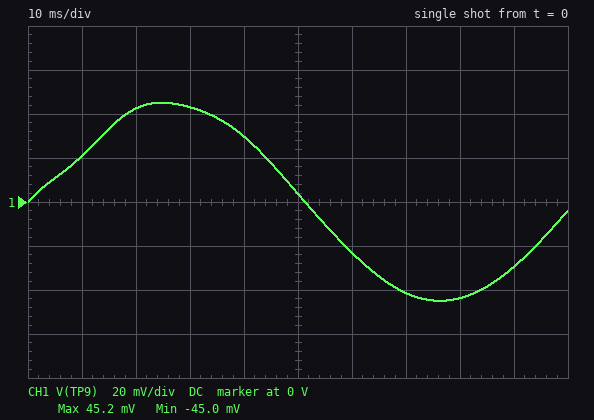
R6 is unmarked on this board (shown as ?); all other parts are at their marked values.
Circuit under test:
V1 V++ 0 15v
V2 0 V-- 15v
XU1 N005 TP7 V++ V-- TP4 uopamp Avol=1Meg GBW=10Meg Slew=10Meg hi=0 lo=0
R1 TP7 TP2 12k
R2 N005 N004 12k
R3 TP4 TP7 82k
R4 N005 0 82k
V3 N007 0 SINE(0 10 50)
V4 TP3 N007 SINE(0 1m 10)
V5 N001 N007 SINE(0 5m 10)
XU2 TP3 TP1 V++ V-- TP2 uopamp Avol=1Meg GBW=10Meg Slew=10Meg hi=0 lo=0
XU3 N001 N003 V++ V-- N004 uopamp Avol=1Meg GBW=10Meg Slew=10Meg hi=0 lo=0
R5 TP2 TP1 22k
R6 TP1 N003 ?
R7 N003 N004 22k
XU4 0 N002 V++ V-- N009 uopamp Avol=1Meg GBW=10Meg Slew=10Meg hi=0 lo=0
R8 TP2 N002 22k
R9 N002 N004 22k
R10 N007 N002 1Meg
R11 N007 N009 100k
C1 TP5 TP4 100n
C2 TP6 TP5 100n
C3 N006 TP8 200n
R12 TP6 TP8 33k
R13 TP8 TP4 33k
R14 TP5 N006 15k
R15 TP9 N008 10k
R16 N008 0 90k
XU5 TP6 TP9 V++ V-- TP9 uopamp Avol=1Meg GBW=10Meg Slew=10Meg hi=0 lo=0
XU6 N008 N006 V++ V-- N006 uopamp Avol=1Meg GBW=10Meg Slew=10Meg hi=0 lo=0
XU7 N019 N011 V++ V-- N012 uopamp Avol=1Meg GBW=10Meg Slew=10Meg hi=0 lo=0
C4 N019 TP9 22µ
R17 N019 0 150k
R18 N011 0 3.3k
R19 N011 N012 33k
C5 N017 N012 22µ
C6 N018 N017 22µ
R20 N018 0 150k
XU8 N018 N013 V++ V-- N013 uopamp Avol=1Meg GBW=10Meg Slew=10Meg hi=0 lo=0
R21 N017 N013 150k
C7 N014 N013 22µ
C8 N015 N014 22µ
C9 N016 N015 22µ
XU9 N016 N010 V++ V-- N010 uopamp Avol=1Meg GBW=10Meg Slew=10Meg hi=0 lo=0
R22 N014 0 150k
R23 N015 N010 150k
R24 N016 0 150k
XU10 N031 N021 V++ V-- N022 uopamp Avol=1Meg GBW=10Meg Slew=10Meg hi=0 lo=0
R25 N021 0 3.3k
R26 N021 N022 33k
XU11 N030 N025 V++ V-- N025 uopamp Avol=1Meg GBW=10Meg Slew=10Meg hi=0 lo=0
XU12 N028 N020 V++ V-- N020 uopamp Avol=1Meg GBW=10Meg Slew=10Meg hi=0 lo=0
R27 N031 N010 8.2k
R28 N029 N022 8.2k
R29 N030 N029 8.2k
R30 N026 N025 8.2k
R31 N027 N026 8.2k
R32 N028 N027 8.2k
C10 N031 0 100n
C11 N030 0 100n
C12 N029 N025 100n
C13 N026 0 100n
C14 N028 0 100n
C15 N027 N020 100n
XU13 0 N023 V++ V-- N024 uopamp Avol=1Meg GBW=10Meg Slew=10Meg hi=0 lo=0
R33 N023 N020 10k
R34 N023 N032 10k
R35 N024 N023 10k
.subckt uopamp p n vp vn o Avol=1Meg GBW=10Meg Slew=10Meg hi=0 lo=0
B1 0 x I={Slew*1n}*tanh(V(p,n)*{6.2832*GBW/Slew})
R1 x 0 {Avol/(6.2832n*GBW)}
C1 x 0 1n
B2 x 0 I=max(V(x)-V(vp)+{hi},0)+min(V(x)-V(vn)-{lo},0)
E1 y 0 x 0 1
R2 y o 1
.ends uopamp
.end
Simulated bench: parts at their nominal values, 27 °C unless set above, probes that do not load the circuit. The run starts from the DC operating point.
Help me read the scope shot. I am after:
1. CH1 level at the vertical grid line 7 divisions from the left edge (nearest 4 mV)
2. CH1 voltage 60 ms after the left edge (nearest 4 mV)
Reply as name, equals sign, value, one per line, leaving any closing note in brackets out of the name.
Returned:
CH1 level at the vertical grid line 7 divisions from the left edge = -40 mV
CH1 voltage 60 ms after the left edge = -24 mV
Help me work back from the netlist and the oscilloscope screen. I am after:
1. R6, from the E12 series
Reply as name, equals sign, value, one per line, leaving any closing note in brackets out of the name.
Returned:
R6, from the E12 series = 68 kΩ
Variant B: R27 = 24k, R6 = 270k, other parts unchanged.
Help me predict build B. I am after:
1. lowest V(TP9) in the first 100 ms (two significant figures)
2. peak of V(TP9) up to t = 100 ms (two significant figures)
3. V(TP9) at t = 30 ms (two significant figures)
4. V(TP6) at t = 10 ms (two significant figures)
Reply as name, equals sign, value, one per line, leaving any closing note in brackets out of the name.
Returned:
lowest V(TP9) in the first 100 ms = -32 mV
peak of V(TP9) up to t = 100 ms = 32 mV
V(TP9) at t = 30 ms = 30 mV
V(TP6) at t = 10 ms = 15 mV
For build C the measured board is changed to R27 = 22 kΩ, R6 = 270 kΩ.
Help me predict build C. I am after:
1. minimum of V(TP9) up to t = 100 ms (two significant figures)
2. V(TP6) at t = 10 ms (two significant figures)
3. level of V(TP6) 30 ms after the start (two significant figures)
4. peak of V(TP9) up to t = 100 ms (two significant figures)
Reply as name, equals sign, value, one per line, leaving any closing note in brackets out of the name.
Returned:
minimum of V(TP9) up to t = 100 ms = -32 mV
V(TP6) at t = 10 ms = 15 mV
level of V(TP6) 30 ms after the start = 30 mV
peak of V(TP9) up to t = 100 ms = 32 mV
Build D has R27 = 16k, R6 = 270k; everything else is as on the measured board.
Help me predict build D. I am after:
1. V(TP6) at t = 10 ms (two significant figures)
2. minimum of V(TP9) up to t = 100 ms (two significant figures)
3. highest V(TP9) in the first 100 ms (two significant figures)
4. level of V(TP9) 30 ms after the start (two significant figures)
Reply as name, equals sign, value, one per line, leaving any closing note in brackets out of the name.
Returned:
V(TP6) at t = 10 ms = 15 mV
minimum of V(TP9) up to t = 100 ms = -32 mV
highest V(TP9) in the first 100 ms = 32 mV
level of V(TP9) 30 ms after the start = 30 mV
